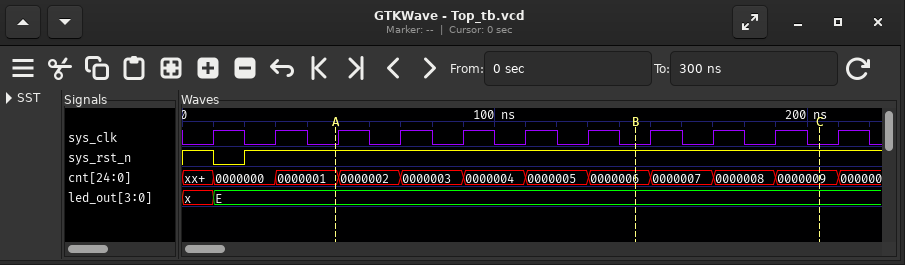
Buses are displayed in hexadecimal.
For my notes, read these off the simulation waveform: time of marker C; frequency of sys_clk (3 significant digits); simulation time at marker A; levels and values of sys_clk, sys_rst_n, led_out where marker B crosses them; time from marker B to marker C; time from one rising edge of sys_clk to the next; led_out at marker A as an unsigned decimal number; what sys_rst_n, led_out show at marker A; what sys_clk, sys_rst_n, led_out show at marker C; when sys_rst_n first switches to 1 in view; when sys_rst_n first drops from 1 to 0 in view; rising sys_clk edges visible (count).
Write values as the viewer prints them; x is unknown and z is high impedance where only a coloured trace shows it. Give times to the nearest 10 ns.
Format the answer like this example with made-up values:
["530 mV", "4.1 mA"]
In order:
["200 ns", "50.0 MHz", "50 ns", "sys_clk=0, sys_rst_n=1, led_out=E", "60 ns", "20 ns", "14", "sys_rst_n=1, led_out=E", "sys_clk=0, sys_rst_n=1, led_out=E", "20 ns", "10 ns", "11"]
